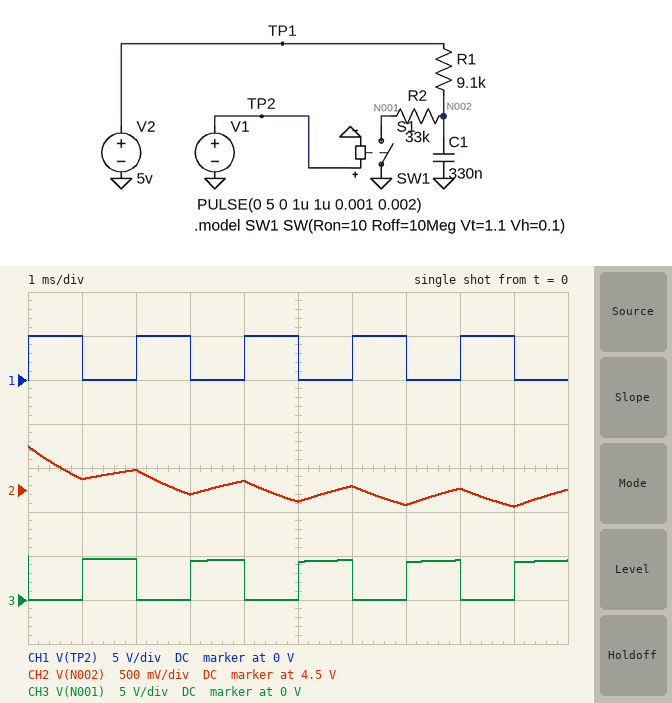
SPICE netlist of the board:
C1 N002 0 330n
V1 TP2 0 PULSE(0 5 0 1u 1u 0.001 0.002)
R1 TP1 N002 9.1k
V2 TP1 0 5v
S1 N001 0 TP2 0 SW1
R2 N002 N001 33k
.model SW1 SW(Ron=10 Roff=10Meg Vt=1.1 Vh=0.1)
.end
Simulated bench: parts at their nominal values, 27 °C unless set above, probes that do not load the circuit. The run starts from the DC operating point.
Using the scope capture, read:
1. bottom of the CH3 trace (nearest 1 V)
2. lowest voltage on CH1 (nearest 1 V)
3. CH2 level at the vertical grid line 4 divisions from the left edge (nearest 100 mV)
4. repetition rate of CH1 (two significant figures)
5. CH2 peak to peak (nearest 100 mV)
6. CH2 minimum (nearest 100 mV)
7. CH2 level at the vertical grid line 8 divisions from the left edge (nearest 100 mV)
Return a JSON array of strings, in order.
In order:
["0 V", "0 V", "4.6 V", "500 Hz", "700 mV", "4.3 V", "4.5 V"]
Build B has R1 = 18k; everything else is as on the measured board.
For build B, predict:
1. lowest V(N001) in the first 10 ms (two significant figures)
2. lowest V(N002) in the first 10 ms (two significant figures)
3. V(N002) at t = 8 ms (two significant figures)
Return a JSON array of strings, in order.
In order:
["1.2 mV", "4.0 V", "4.2 V"]
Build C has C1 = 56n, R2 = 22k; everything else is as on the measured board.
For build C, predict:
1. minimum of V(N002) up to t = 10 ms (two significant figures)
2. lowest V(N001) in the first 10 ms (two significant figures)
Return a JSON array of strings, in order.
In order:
["3.6 V", "1.6 mV"]
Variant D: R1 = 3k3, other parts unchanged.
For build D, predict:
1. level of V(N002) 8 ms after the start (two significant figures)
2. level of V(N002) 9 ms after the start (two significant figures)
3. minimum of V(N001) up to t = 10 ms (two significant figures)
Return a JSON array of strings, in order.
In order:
["4.9 V", "4.7 V", "1.4 mV"]
